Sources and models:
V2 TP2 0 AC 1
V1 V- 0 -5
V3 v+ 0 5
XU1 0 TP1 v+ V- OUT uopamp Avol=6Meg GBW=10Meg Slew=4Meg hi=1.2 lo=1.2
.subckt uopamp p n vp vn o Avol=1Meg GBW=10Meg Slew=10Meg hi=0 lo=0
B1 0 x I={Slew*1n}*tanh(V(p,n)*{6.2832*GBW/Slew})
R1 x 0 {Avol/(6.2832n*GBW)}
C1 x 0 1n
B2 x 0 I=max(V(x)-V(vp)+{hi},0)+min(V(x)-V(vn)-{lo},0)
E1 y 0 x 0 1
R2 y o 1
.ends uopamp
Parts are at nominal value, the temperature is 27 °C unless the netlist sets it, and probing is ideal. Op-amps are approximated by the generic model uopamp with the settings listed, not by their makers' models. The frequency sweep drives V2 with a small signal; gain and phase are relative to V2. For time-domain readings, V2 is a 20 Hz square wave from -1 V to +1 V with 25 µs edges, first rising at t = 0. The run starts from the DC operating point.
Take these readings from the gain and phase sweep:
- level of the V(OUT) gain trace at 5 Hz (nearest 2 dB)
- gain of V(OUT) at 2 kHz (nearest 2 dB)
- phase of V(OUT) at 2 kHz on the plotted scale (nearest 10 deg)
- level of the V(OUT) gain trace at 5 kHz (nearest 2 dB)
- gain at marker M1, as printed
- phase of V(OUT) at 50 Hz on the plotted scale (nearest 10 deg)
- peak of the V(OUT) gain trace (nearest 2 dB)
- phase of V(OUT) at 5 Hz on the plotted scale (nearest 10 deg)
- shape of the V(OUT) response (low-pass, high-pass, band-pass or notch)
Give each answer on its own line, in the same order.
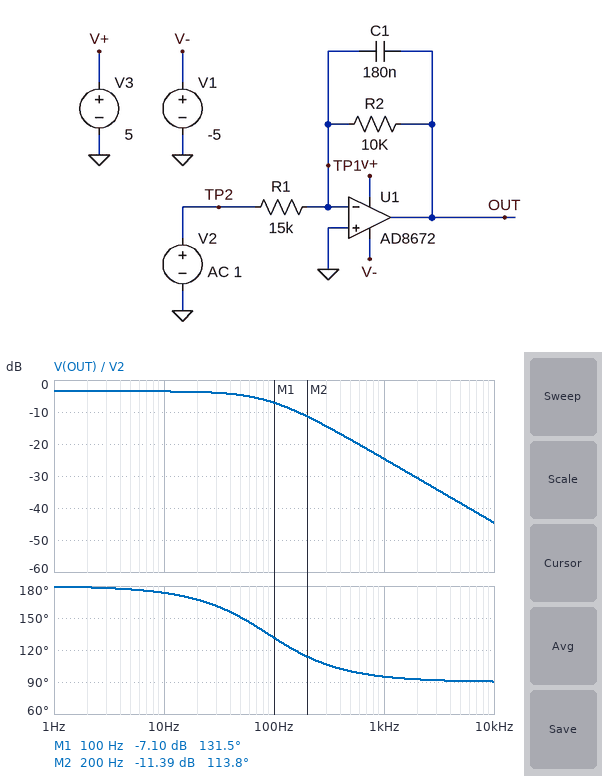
-4 dB
-30 dB
90 deg
-38 dB
-7.10 dB
150 deg
-4 dB
180 deg
low-pass
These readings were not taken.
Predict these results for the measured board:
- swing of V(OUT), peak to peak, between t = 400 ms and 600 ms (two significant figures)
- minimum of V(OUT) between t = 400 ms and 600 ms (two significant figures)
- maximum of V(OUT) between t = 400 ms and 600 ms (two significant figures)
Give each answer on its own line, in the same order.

1.3 V
-670 mV
670 mV
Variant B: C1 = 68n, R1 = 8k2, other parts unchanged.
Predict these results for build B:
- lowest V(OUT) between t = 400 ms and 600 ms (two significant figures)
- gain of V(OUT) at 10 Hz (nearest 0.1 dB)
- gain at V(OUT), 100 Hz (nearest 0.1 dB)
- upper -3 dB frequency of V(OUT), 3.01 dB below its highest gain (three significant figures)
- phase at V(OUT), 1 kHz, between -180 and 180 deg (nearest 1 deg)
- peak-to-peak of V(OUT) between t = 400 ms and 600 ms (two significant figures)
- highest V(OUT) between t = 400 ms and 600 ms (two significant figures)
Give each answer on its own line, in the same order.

-1.2 V
1.7 dB
1.0 dB
234 Hz
103 deg
2.4 V
1.2 V
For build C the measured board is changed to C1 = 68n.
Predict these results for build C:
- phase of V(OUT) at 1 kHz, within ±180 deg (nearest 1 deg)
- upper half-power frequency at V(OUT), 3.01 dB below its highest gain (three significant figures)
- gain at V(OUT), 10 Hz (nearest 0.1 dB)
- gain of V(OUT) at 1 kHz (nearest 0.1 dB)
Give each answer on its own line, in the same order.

103 deg
234 Hz
-3.5 dB
-16.4 dB
